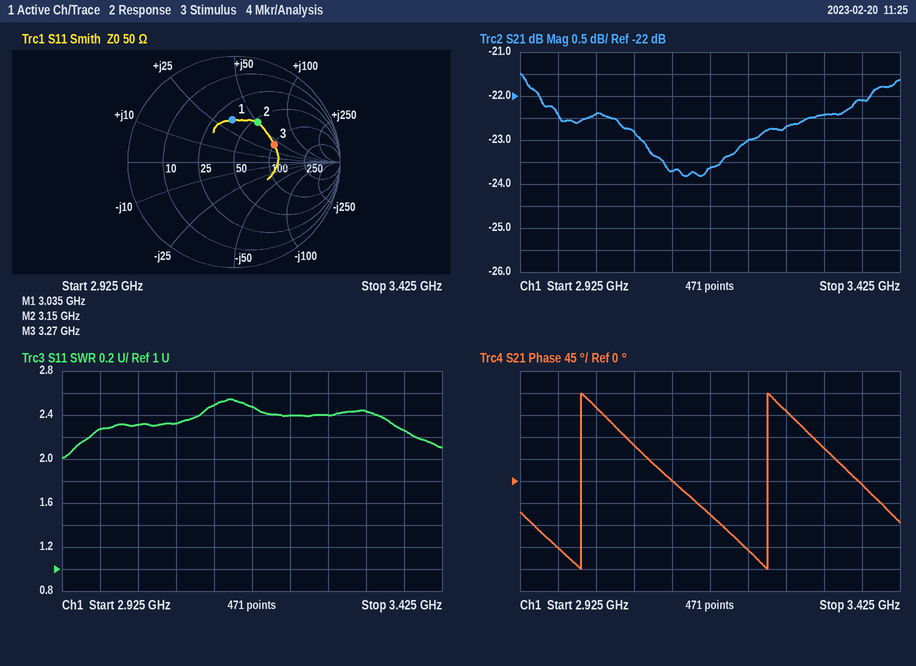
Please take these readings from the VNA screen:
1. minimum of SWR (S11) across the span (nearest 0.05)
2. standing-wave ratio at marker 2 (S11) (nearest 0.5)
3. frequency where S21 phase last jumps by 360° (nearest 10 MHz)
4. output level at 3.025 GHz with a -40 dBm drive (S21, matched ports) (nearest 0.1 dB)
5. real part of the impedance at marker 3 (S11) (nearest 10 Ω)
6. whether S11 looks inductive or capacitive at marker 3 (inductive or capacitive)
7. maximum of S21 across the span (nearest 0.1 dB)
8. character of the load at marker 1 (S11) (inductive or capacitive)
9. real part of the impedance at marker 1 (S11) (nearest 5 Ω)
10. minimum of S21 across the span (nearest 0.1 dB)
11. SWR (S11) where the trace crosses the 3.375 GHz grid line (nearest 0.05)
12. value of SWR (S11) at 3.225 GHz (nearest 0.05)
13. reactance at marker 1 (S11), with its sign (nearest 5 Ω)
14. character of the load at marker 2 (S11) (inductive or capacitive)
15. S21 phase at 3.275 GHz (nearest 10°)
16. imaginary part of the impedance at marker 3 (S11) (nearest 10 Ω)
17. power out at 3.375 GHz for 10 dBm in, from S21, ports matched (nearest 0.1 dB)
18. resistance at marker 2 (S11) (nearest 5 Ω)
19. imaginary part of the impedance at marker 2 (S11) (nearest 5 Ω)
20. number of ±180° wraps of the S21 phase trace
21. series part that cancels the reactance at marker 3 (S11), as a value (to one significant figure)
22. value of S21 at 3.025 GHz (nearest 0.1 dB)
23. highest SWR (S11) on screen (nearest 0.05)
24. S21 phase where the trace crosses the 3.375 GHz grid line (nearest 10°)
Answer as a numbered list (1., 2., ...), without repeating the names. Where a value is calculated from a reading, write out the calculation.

1. 2.00
2. 2.5
3. 3.25 GHz
4. -40 dBm + (-22.4 dB) = -62.4 dBm
5. 100 Ω
6. inductive
7. -21.5 dB
8. inductive
9. 35 Ω
10. -23.8 dB
11. 2.25
12. 2.40
13. +35 Ω
14. inductive
15. 140°
16. +40 Ω
17. 10 dBm + (-22.1 dB) = -12.1 dBm
18. 55 Ω
19. +50 Ω
20. 2
21. C = 1/(2π × 3.27 GHz × 40 Ω) ≈ 1 pF
22. -22.4 dB
23. 2.55
24. -10°
